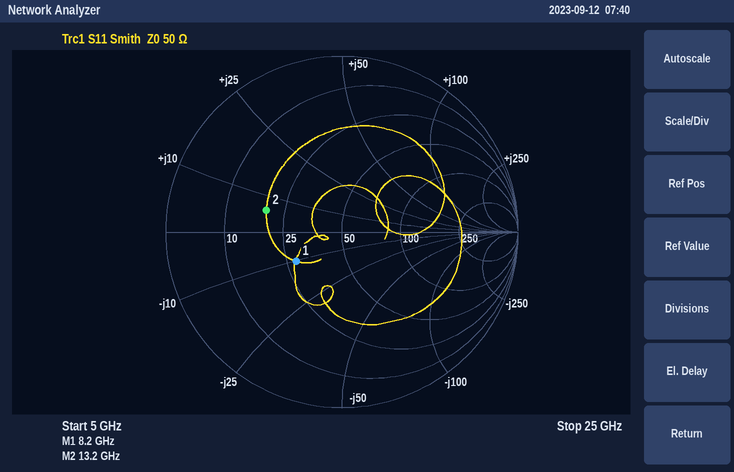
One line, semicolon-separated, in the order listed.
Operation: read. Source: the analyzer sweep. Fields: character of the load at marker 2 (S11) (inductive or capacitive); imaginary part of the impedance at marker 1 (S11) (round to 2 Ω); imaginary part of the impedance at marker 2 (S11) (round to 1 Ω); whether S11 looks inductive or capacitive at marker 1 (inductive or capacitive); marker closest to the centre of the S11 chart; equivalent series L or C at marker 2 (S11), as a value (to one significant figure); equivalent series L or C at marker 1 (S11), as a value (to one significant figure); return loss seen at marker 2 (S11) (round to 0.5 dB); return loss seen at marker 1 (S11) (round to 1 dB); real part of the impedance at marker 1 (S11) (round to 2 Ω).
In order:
inductive; -10 Ω; +6 Ω; capacitive; marker 1; 70 pH; 2 pF; 7.0 dB; 10 dB; 28 Ω
